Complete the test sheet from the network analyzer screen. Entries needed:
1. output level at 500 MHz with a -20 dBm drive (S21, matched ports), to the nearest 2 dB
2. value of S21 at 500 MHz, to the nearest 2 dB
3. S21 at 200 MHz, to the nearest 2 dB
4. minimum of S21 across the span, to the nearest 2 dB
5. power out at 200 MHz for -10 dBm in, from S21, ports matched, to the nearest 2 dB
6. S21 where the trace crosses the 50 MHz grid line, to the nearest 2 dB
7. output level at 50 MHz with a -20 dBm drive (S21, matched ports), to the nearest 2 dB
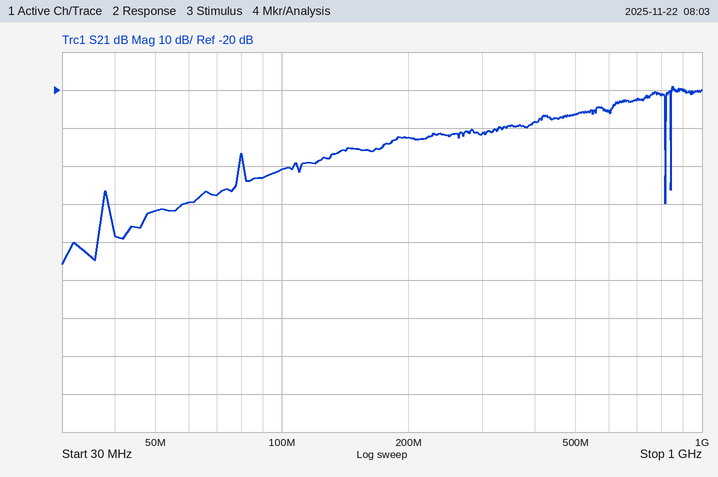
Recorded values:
-46 dBm
-26 dB
-32 dB
-66 dB
-42 dBm
-52 dB
-72 dBm
